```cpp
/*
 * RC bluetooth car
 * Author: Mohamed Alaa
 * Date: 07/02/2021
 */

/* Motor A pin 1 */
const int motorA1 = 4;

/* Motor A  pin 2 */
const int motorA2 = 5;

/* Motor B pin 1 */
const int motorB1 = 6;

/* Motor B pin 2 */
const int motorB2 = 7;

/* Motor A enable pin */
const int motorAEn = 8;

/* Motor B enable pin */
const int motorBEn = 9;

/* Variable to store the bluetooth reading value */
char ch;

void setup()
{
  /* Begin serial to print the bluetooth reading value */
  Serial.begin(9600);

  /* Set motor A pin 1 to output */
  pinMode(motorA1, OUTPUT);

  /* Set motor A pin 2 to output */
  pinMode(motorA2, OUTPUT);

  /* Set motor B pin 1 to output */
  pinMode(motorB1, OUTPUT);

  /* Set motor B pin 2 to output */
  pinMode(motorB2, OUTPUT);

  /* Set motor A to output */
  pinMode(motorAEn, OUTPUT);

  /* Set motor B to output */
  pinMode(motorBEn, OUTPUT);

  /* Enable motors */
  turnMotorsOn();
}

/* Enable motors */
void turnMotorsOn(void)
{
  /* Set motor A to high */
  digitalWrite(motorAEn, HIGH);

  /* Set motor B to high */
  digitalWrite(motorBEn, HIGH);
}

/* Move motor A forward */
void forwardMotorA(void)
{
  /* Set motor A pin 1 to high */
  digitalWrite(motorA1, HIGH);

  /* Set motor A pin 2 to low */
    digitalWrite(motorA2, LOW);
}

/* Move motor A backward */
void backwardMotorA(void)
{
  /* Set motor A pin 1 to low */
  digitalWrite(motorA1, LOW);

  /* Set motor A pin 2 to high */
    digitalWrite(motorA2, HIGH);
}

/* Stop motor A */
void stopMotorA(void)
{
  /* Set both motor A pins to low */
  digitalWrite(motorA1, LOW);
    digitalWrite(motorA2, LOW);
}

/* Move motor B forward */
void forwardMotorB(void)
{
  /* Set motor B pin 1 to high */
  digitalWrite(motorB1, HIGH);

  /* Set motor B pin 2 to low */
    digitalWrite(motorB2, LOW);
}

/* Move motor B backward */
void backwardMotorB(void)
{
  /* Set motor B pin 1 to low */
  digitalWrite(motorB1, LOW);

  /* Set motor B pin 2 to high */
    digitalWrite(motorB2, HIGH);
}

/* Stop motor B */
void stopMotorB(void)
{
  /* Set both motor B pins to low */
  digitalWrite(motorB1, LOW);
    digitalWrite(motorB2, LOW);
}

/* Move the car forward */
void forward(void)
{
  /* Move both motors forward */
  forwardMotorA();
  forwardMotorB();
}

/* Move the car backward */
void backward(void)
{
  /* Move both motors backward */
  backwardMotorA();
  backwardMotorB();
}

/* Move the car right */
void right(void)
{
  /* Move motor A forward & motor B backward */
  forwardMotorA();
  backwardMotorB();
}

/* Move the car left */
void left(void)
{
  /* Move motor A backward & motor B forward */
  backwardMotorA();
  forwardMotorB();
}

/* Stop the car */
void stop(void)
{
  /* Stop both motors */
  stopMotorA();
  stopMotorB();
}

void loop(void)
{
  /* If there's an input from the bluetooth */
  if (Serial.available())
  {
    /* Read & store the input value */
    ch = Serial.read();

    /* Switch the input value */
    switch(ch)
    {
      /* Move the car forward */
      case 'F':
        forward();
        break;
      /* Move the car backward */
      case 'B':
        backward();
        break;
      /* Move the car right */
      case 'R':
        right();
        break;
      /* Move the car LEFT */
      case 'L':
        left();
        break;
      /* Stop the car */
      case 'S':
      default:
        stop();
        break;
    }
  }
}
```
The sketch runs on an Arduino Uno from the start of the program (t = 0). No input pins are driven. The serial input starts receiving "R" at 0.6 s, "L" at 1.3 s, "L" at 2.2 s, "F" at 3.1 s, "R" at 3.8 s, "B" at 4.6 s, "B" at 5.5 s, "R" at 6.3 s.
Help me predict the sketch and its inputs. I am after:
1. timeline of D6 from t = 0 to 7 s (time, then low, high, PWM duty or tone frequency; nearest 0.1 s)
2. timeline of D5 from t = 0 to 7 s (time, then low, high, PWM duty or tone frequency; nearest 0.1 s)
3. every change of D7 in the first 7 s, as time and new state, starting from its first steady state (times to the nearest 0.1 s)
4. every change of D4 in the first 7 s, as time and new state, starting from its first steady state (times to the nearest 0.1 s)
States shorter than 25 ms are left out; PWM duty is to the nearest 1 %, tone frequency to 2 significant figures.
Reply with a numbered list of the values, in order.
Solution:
1. 0 s low; 1.3 s high; 3.8 s low
2. 0 s low; 1.3 s high; 3.1 s low; 4.6 s high; 6.3 s low
3. 0 s low; 0.6 s high; 1.3 s low; 3.8 s high
4. 0 s low; 0.6 s high; 1.3 s low; 3.1 s high; 4.6 s low; 6.3 s high
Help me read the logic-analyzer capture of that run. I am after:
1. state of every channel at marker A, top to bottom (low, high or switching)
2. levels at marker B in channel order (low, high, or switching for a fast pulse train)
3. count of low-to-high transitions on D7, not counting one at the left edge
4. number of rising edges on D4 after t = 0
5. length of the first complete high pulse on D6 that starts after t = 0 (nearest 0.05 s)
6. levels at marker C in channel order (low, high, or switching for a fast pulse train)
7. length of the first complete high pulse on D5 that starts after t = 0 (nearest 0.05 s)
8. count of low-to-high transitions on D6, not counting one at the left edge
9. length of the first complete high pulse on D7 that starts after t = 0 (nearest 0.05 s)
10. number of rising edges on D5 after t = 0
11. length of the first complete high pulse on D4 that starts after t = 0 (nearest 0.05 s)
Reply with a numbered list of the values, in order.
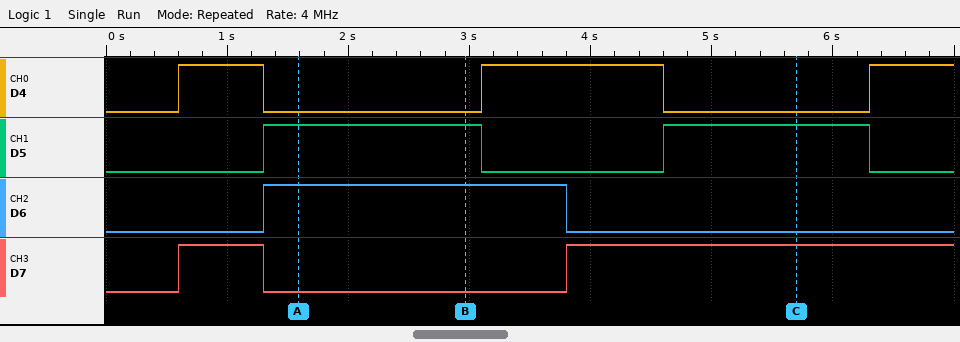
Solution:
1. D4 low, D5 high, D6 high, D7 low
2. D4 low, D5 high, D6 high, D7 low
3. 2
4. 3
5. 2.50 s
6. D4 low, D5 high, D6 low, D7 high
7. 1.80 s
8. 1
9. 0.70 s
10. 2
11. 0.70 s
